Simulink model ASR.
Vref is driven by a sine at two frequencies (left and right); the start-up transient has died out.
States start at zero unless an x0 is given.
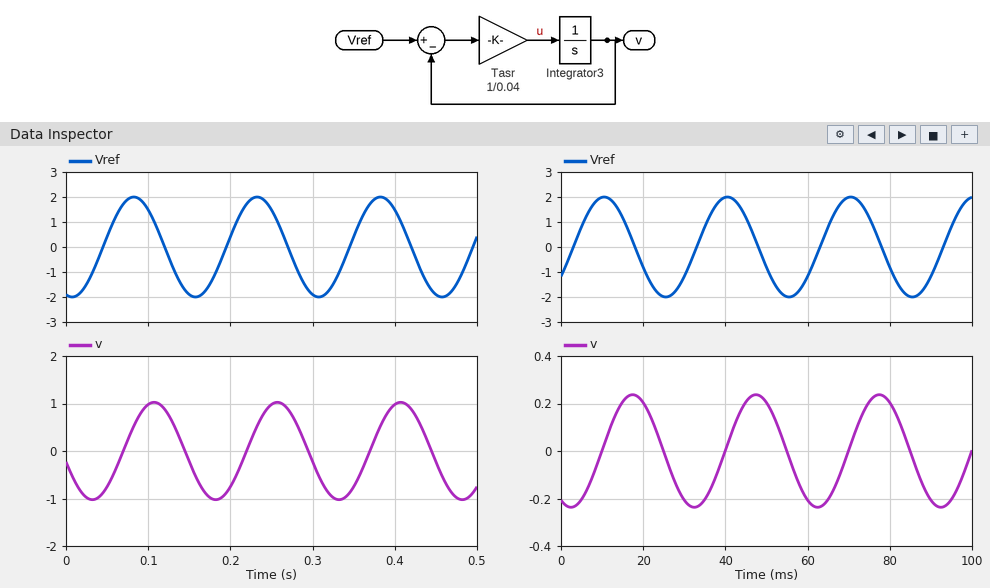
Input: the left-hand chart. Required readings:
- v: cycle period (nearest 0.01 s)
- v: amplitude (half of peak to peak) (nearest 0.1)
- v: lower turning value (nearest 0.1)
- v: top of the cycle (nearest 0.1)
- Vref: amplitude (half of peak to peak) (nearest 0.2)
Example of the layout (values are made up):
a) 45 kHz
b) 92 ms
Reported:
a) 0.15 s
b) 1.0
c) -1.0
d) 1.0
e) 2.0
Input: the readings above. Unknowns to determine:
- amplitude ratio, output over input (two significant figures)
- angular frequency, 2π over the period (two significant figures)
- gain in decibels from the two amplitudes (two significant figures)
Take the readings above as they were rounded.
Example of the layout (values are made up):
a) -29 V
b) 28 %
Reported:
a) 0.50
b) 42 rad/s
c) -6.0 dB
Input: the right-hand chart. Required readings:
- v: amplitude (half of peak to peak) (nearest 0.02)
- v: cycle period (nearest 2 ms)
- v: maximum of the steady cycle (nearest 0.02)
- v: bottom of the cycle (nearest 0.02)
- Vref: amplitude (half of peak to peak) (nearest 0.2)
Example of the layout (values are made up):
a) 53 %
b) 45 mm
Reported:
a) 0.24
b) 30 ms
c) 0.24
d) -0.24
e) 2.0
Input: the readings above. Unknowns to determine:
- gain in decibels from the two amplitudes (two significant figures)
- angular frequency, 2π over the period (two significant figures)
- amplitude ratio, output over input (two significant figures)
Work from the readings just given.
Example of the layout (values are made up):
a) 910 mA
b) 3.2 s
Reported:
a) -18 dB
b) 0.21 rad/ms
c) 0.12
